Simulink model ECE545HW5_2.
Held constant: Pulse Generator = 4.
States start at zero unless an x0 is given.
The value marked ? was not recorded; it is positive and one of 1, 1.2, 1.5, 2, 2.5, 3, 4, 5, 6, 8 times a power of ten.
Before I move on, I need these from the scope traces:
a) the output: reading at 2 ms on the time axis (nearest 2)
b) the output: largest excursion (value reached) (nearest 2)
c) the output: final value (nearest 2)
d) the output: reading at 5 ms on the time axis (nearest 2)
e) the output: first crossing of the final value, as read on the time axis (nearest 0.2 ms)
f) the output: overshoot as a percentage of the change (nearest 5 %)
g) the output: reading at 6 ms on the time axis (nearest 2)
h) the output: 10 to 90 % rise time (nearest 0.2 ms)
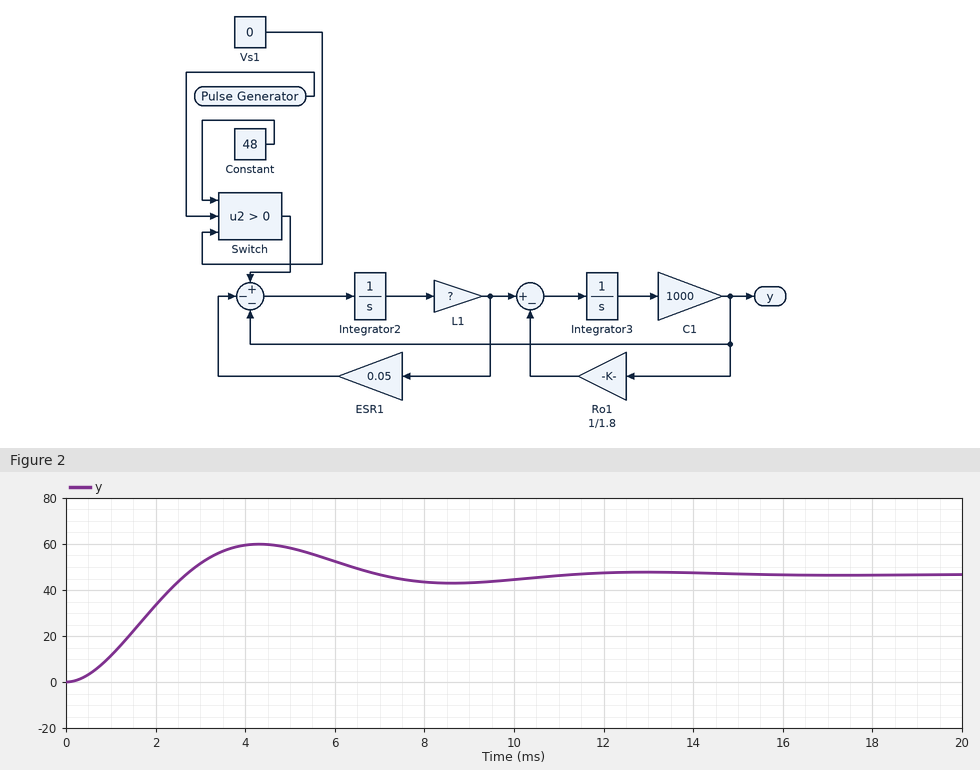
34
60
46
58
2.6 ms
30 %
52
1.8 ms
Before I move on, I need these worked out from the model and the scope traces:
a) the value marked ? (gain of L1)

600
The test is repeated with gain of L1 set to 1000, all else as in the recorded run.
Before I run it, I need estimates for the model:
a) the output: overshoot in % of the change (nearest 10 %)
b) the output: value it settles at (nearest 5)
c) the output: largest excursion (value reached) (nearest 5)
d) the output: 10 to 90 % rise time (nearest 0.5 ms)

40 %
45
65
1.5 ms
